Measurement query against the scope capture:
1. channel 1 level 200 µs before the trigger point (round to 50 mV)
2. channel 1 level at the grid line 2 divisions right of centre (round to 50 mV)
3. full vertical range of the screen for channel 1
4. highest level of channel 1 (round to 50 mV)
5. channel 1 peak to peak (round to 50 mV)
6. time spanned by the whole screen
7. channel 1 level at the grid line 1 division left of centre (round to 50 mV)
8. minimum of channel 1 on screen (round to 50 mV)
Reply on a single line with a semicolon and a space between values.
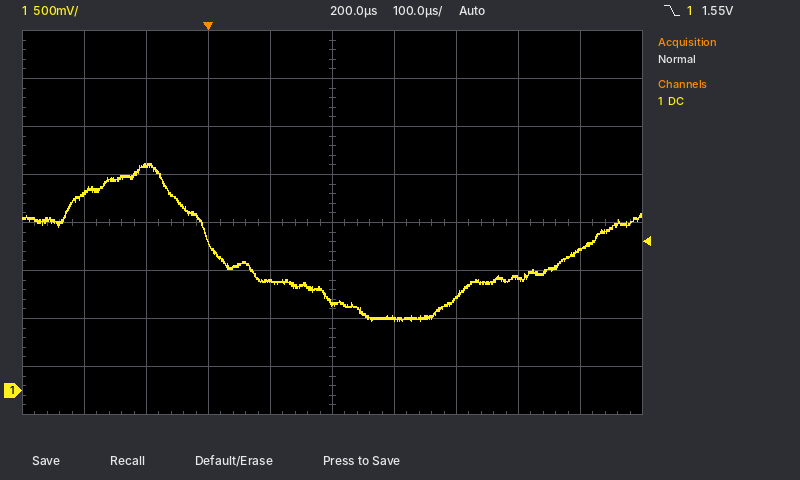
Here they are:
2.05 V; 950 mV; 4 V; 2.35 V; 1.65 V; 1 ms; 1.15 V; 700 mV
